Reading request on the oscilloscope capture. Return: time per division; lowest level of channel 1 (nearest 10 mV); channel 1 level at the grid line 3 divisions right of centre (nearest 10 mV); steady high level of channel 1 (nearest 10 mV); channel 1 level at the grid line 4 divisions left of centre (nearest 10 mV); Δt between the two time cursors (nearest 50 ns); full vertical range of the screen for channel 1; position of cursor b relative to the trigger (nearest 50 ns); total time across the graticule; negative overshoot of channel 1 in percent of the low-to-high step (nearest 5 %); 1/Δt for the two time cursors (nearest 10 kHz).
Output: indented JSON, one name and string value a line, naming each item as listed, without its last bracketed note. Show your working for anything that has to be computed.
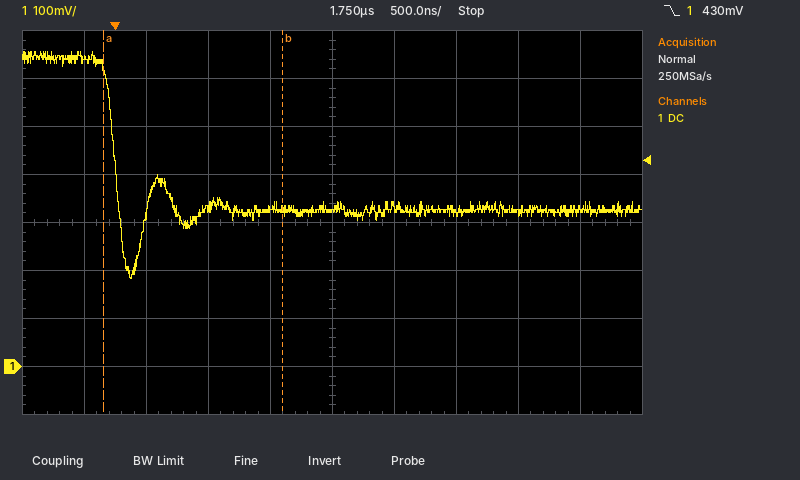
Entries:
{
  "time per division": "500 ns",
  "lowest level of channel 1": "180 mV",
  "channel 1 level at the grid line 3 divisions right of centre": "320 mV",
  "steady high level of channel 1": "640 mV",
  "channel 1 level at the grid line 4 divisions left of centre": "640 mV",
  "Δt between the two time cursors": "1.45 µs",
  "full vertical range of the screen for channel 1": "800 mV",
  "position of cursor b relative to the trigger": "+1.35 µs",
  "total time across the graticule": "5 µs",
  "negative overshoot of channel 1 in percent of the low-to-high step": "45 %",
  "1/Δt for the two time cursors": "1 / 1.45 µs ≈ 690 kHz"
}
